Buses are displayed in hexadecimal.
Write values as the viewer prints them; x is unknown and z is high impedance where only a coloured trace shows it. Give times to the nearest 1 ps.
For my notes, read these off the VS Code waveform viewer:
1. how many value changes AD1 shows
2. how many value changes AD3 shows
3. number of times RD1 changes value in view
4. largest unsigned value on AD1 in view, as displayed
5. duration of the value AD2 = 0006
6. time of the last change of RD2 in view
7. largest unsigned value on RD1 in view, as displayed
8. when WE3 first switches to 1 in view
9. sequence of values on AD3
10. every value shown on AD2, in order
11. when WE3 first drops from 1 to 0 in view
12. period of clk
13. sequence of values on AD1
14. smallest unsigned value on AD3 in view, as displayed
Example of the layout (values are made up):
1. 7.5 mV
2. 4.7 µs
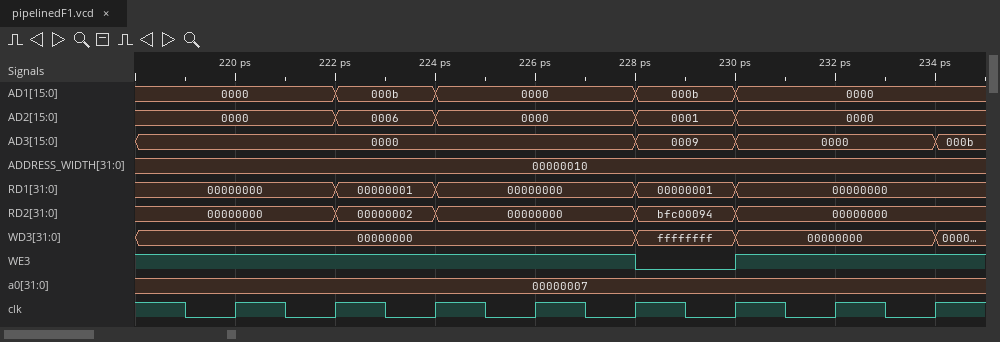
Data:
1. 4
2. 3
3. 4
4. 000b
5. 2 ps
6. 230 ps
7. 00000001
8. 230 ps
9. 0000, 0009, 0000, 000b
10. 0000, 0006, 0000, 0001, 0000
11. 228 ps
12. 2 ps
13. 0000, 000b, 0000, 000b, 0000
14. 0000
